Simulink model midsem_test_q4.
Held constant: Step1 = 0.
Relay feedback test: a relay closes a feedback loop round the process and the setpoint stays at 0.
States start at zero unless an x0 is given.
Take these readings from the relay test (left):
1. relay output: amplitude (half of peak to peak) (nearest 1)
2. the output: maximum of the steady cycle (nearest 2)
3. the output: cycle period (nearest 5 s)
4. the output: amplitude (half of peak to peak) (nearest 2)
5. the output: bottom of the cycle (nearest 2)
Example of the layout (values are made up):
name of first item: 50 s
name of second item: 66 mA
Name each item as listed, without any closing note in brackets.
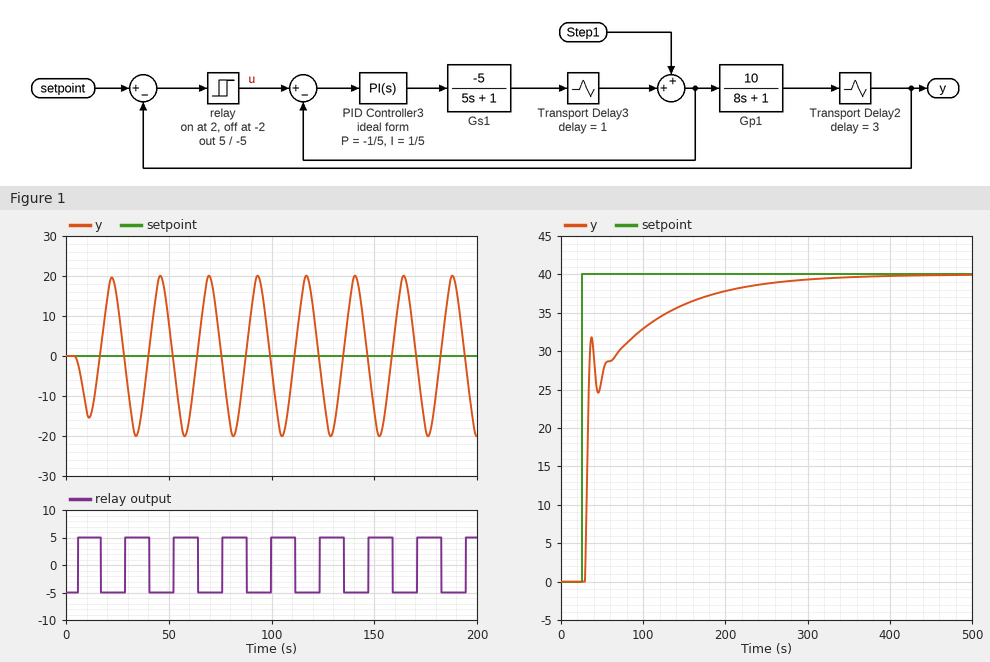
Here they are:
relay output: amplitude (half of peak to peak): 5
the output: maximum of the steady cycle: 20
the output: cycle period: 25 s
the output: amplitude (half of peak to peak): 20
the output: bottom of the cycle: -20
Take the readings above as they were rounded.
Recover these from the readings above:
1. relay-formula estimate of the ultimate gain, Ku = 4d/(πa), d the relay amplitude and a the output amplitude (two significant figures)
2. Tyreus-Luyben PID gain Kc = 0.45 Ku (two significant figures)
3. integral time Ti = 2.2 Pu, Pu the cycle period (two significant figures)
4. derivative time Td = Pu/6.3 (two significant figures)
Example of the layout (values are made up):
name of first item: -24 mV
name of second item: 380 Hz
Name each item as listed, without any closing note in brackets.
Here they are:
relay-formula estimate of the ultimate gain, Ku = 4d/(πa), d the relay amplitude and a the output amplitude: 0.32
Tyreus-Luyben PID gain Kc = 0.45 Ku: 0.14
integral time Ti = 2.2 Pu, Pu the cycle period: 55 s
derivative time Td = Pu/6.3: 4.0 s
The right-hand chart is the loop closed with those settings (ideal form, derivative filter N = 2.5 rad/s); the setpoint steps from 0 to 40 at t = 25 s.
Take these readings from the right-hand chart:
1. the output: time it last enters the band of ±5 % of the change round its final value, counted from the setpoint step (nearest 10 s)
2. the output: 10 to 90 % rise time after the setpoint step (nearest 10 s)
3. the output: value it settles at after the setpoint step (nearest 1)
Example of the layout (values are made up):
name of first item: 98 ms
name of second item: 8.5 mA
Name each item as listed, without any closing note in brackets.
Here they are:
the output: time it last enters the band of ±5 % of the change round its final value, counted from the setpoint step: 180 s
the output: 10 to 90 % rise time after the setpoint step: 120 s
the output: value it settles at after the setpoint step: 40
